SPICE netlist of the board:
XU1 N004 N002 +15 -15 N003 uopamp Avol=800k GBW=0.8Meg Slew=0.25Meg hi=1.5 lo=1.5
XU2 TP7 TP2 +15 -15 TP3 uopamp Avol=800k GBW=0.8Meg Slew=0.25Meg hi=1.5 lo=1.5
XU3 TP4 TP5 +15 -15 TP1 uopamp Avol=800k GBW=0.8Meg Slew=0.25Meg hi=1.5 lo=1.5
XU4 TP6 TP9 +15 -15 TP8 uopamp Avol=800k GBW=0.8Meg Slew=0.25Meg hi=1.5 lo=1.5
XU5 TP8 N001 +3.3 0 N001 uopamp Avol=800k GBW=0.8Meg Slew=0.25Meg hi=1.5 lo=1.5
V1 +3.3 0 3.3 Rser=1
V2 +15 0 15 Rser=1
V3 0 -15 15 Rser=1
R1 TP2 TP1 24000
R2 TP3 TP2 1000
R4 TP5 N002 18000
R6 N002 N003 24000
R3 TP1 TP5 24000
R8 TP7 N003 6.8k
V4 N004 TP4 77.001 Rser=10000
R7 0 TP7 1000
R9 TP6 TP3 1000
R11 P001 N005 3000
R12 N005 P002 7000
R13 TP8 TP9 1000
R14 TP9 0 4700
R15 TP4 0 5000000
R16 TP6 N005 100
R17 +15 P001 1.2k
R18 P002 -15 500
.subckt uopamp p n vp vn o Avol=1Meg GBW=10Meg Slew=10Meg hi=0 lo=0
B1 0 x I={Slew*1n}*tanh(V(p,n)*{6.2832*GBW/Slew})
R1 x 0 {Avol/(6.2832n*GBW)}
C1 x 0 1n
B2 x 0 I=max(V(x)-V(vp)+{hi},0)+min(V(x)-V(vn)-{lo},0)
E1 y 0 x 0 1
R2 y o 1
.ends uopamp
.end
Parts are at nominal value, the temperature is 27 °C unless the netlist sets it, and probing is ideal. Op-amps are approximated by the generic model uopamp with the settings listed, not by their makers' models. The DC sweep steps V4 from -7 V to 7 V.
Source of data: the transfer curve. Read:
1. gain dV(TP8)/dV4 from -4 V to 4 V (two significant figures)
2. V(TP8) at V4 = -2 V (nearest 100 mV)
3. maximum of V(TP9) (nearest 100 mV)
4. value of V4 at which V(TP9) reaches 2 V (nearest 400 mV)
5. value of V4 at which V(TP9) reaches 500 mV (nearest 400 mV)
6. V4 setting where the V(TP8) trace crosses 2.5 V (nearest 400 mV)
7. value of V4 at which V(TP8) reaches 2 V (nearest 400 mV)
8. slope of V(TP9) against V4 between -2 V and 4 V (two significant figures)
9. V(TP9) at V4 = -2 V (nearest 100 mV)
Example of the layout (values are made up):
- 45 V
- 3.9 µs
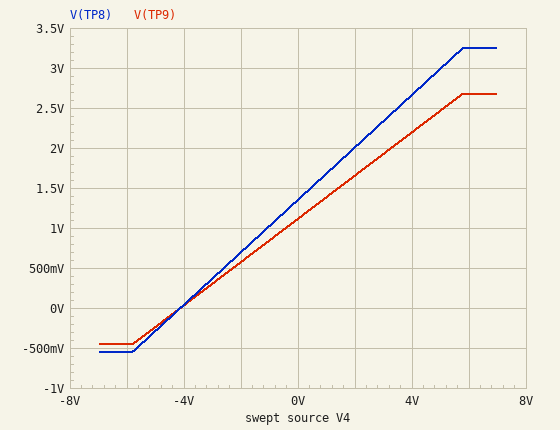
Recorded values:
- 0.33 V/V
- 700 mV
- 2.7 V
- 3.2 V
- -2.4 V
- 3.6 V
- 2.0 V
- 0.27 V/V
- 600 mV
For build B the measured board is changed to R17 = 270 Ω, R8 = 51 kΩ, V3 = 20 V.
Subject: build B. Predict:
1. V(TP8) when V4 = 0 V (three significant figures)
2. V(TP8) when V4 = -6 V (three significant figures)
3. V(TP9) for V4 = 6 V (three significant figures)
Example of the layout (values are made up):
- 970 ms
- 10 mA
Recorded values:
- 1.57 V
- 1.05 V
- 1.71 V
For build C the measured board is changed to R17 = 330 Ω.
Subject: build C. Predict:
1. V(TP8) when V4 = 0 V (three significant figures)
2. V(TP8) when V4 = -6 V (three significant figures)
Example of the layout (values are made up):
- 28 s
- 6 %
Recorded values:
- 2.06 V
- 236 mV
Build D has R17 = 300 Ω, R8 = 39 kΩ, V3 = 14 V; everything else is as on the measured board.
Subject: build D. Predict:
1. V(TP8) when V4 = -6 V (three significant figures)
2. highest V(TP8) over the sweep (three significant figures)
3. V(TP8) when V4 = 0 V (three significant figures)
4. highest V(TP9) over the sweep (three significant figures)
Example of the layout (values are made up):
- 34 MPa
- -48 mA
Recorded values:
- 1.66 V
- 2.77 V
- 2.19 V
- 2.28 V
